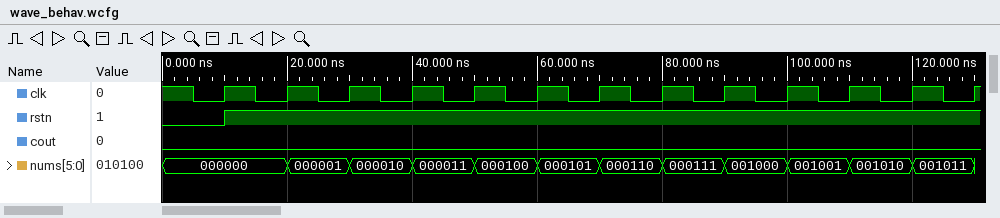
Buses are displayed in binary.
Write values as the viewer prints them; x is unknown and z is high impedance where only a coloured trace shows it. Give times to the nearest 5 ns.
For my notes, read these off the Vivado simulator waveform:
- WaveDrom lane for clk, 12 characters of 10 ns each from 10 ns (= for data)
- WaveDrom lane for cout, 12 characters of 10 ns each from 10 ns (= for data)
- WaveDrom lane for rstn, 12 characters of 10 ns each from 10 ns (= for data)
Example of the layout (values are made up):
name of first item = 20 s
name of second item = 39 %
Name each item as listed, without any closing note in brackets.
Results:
WaveDrom lane for clk, 12 characters of 10 ns each from 10 ns = {name: 'clk', wave: 'p...........'}
WaveDrom lane for cout, 12 characters of 10 ns each from 10 ns = {name: 'cout', wave: '0...........'}
WaveDrom lane for rstn, 12 characters of 10 ns each from 10 ns = {name: 'rstn', wave: '1...........'}
